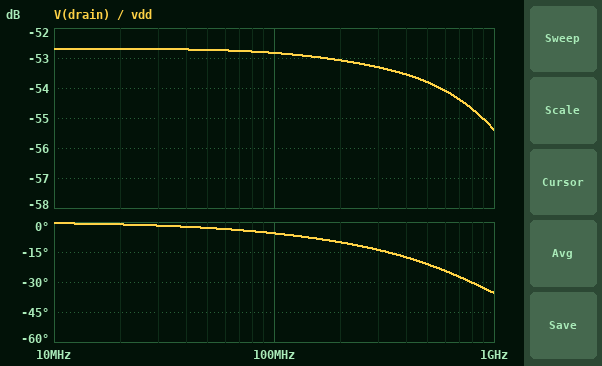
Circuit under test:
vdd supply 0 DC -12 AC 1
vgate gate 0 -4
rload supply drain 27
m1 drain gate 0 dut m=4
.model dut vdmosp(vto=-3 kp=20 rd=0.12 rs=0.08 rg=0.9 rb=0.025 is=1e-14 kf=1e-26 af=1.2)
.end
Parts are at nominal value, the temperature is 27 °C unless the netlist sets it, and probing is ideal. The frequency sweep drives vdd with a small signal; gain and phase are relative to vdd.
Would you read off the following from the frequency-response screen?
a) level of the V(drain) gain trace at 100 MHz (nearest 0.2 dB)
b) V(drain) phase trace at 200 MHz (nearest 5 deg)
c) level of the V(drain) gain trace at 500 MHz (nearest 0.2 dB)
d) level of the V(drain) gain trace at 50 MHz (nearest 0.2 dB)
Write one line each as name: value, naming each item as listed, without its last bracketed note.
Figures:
level of the V(drain) gain trace at 100 MHz: -52.8 dB
V(drain) phase trace at 200 MHz: -10 deg
level of the V(drain) gain trace at 500 MHz: -53.8 dB
level of the V(drain) gain trace at 50 MHz: -52.8 dB
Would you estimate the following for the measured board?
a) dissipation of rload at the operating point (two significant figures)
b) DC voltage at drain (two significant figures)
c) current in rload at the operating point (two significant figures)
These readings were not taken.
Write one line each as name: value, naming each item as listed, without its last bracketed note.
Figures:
dissipation of rload at the operating point: 5.3 W
DC voltage at drain: -28 mV
current in rload at the operating point: 440 mA
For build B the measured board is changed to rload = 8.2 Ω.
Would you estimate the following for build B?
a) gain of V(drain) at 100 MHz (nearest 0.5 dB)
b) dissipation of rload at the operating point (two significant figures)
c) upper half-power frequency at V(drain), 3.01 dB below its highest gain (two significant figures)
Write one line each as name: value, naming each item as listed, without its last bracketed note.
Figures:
gain of V(drain) at 100 MHz: -42.5 dB
dissipation of rload at the operating point: 17 W
upper half-power frequency at V(drain), 3.01 dB below its highest gain: 1.1 GHz
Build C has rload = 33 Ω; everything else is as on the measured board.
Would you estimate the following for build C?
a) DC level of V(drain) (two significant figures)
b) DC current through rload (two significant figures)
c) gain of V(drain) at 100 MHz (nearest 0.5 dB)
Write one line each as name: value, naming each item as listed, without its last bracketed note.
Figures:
DC level of V(drain): -23 mV
DC current through rload: 360 mA
gain of V(drain) at 100 MHz: -54.5 dB
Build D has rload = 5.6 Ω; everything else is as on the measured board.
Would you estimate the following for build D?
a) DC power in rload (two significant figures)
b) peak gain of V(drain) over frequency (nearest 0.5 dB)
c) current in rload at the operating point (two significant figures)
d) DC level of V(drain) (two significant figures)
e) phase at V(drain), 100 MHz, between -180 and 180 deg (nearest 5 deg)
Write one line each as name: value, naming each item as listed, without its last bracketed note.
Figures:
DC power in rload: 25 W
peak gain of V(drain) over frequency: -39.0 dB
current in rload at the operating point: 2.1 A
DC level of V(drain): -130 mV
phase at V(drain), 100 MHz, between -180 and 180 deg: -5 deg
